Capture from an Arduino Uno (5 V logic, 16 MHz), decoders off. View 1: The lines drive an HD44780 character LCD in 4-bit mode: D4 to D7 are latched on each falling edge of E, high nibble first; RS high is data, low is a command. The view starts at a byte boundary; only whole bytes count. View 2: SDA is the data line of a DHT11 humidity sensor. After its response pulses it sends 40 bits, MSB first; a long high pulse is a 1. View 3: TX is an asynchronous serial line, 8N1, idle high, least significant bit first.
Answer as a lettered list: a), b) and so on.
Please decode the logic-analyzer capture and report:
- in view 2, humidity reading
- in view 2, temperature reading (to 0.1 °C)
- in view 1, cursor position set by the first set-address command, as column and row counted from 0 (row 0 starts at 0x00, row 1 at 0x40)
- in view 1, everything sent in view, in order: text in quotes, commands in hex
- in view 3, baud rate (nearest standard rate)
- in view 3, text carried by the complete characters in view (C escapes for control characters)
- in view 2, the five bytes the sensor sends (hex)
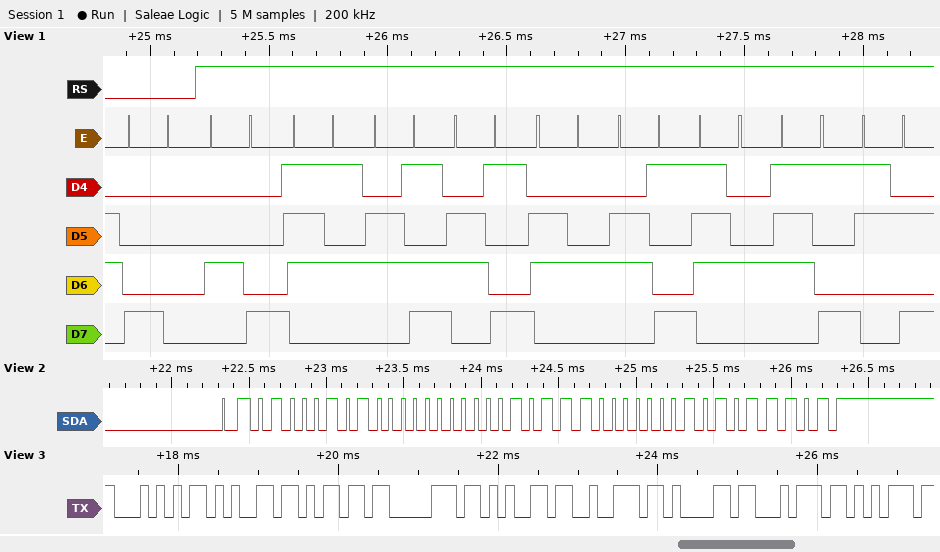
a) 69 %
b) 23.1 °C
c) column 0, row 0
d) 0x80 "Humidity:"
e) 9600 baud
f) "Temperatu"
g) 45 00 17 01 5D
